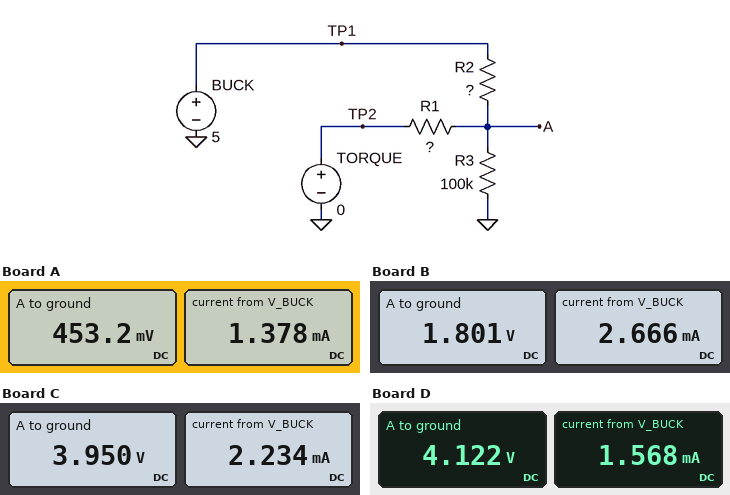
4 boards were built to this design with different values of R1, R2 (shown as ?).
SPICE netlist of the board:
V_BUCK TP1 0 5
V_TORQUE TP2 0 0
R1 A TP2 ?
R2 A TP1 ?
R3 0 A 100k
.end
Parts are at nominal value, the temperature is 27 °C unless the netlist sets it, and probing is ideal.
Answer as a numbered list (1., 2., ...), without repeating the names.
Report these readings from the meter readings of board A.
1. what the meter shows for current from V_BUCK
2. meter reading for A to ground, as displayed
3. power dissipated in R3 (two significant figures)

1. 1.378 mA
2. 453.2 mV
3. 2.1 µW
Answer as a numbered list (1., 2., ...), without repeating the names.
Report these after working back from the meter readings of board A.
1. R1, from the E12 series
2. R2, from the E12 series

1. 330 Ω
2. 3.3 kΩ
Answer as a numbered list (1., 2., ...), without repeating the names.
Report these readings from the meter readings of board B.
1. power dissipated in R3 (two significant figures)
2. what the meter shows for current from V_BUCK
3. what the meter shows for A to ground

1. 32 µW
2. 2.666 mA
3. 1.801 V
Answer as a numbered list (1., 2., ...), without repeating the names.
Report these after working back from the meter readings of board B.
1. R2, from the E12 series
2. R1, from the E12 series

1. 1.2 kΩ
2. 680 Ω
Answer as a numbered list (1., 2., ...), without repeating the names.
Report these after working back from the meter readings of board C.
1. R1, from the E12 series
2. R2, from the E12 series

1. 1.8 kΩ
2. 470 Ω
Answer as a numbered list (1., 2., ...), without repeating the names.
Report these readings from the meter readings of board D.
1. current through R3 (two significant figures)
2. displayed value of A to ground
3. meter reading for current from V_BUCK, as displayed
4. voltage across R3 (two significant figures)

1. 41 µA
2. 4.122 V
3. 1.568 mA
4. 4.1 V
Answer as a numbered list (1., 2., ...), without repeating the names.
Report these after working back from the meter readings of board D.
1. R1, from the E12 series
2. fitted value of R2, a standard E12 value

1. 2.7 kΩ
2. 560 Ω
